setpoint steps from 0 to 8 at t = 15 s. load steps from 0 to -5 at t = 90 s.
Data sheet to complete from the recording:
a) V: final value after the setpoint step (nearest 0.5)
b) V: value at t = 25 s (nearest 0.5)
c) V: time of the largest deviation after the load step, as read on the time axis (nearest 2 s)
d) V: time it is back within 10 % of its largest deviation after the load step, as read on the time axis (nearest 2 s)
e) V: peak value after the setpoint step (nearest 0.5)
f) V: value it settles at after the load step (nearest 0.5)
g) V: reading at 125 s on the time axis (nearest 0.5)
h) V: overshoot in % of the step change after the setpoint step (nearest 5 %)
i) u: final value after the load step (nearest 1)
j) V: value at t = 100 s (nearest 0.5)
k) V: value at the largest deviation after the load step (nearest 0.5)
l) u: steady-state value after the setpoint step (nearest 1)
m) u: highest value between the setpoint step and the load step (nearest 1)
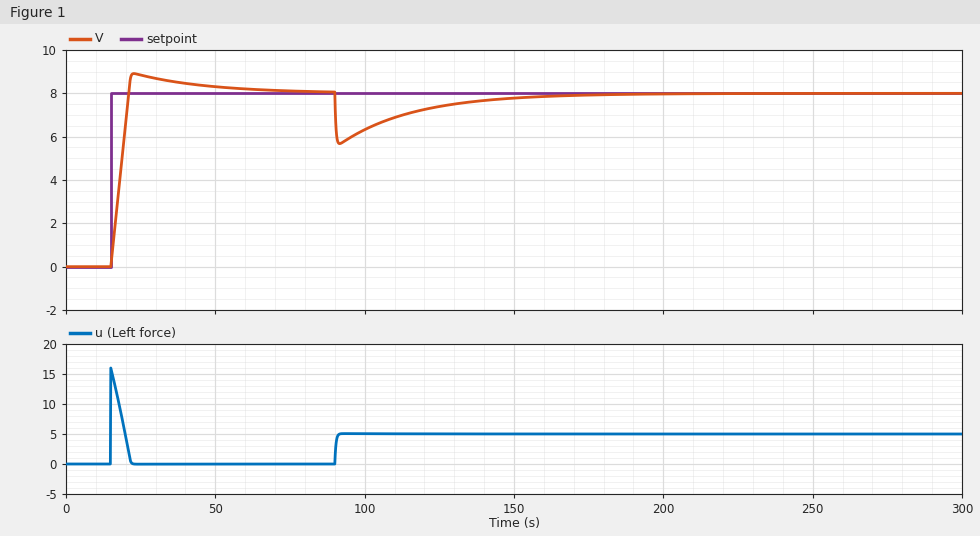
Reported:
8.0
9.0
92 s
148 s
9.0
8.0
7.5
10 %
5
6.5
5.5
0
16
